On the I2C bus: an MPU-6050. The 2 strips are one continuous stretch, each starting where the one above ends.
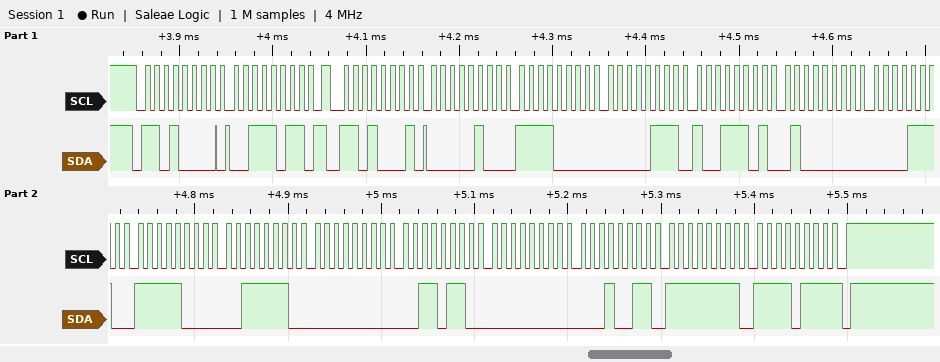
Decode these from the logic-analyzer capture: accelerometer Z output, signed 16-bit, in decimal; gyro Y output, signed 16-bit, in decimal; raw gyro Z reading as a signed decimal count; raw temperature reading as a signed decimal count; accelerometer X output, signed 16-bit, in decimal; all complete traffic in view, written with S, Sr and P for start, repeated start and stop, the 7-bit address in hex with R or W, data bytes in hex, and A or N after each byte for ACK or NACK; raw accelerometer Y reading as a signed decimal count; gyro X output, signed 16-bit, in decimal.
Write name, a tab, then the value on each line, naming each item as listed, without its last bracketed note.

accelerometer Z output, signed 16-bit, in decimal	16398
gyro Y output, signed 16-bit, in decimal	19
raw gyro Z reading as a signed decimal count	-9
raw temperature reading as a signed decimal count	-1986
accelerometer X output, signed 16-bit, in decimal	1264
all complete traffic in view, written with S, Sr and P for start, repeated start and stop, the 7-bit address in hex with R or W, data bytes in hex, and A or N after each byte for ACK or NACK	S 68W A 3B A Sr 68R A 04 A F0 A 07 A 9D A 40 A 0E A F8 A 3E A 00 A 36 A 00 A 13 A FF A F7 N P
raw accelerometer Y reading as a signed decimal count	1949
gyro X output, signed 16-bit, in decimal	54
